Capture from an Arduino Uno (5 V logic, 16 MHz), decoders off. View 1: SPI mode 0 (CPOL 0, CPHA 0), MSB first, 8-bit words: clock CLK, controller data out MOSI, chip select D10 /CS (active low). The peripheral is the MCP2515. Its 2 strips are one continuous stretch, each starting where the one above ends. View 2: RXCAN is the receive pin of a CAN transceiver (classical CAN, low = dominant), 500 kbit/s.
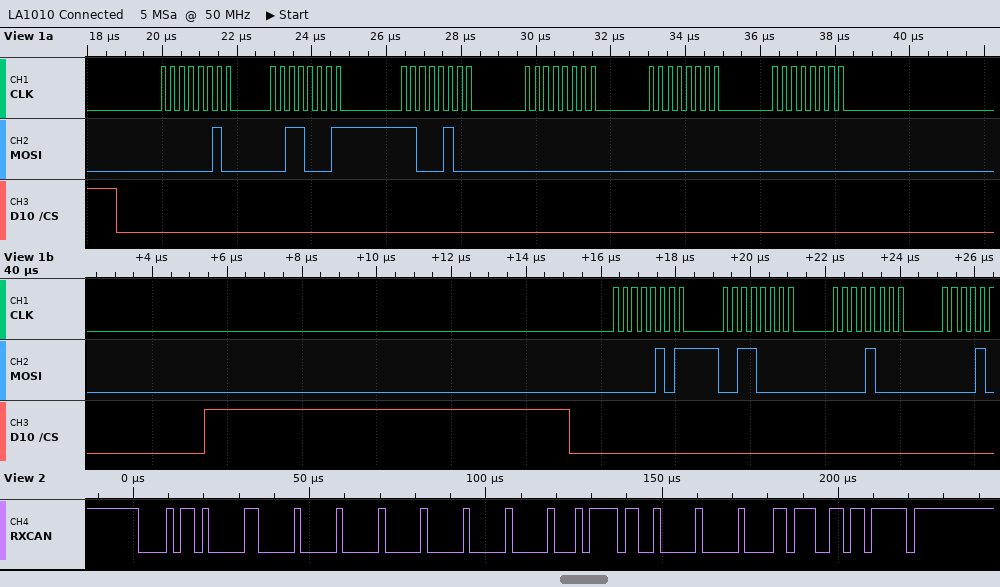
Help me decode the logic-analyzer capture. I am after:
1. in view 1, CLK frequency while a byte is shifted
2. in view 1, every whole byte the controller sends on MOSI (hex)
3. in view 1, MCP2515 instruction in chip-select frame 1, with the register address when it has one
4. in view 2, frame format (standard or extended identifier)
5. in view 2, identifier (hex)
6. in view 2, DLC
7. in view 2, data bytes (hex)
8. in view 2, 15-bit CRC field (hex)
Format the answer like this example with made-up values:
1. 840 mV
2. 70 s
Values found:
1. 4 MHz
2. 0x02 0x31 0xC4 0x00 0x00 0x00 0x05 0x30 0x08
3. WRITE 0x31
4. standard
5. 0x0B4
6. 8
7. 00 00 00 00 17 B2 00 06
8. 0x736F
